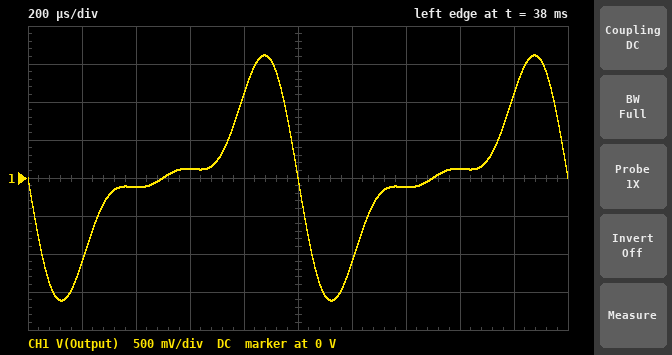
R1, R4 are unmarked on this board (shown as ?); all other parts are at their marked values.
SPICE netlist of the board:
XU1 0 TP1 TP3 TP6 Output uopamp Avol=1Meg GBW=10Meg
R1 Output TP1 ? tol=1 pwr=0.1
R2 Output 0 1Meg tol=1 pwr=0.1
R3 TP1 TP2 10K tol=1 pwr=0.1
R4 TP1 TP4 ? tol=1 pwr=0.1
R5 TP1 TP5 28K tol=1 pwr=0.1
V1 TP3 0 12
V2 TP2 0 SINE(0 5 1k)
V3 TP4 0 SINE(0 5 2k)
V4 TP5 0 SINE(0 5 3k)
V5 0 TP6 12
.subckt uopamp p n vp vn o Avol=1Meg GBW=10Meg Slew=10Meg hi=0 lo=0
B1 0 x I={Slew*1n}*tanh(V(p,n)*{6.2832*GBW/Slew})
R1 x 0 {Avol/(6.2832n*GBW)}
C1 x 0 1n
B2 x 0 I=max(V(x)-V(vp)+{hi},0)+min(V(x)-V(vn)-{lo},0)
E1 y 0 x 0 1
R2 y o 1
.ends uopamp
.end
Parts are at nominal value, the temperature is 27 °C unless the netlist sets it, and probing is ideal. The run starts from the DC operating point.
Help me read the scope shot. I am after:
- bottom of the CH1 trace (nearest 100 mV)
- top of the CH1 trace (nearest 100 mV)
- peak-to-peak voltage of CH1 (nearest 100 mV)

-1.6 V
1.6 V
3.2 V
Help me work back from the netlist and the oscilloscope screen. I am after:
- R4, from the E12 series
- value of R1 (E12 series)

12 kΩ
1.8 kΩ
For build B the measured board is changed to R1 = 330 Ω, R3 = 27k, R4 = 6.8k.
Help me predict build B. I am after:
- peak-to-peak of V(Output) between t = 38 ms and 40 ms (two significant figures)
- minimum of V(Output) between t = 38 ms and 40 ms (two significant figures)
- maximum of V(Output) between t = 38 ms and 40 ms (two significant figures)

660 mV
-330 mV
330 mV
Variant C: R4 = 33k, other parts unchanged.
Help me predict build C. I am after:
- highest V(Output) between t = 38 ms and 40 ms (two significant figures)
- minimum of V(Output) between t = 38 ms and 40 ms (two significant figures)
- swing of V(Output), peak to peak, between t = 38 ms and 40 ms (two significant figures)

1.1 V
-1.1 V
2.3 V
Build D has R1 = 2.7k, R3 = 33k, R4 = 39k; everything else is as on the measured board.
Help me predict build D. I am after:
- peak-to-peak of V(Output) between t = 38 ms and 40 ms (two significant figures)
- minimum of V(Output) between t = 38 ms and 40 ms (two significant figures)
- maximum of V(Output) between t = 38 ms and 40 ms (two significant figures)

2.1 V
-1.0 V
1.0 V
